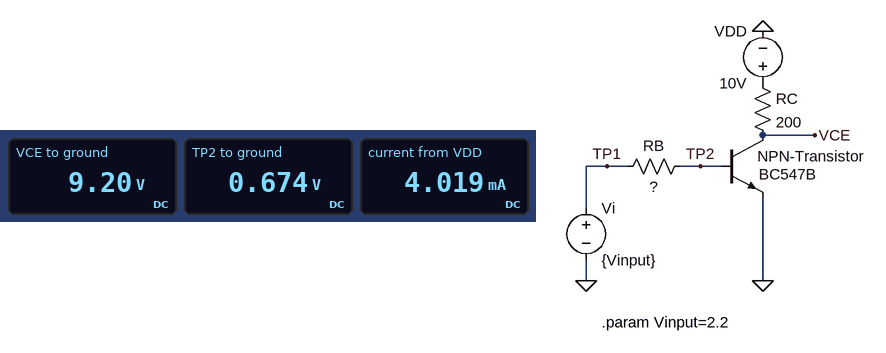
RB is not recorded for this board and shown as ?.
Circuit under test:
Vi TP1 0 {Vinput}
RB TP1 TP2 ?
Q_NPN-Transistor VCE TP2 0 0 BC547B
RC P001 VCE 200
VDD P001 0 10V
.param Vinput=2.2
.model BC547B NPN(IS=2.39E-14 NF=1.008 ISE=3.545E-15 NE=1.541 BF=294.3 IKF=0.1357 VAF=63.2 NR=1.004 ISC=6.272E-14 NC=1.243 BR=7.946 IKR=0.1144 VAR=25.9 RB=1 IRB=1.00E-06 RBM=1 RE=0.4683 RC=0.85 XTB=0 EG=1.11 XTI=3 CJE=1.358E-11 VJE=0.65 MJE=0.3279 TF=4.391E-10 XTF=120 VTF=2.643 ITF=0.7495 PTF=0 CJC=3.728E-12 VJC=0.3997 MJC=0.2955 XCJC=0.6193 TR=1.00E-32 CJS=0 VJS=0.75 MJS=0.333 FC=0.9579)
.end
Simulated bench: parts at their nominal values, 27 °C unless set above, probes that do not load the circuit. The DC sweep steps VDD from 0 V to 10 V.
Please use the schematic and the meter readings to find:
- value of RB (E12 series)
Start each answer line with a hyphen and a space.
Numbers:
- 120 kΩ
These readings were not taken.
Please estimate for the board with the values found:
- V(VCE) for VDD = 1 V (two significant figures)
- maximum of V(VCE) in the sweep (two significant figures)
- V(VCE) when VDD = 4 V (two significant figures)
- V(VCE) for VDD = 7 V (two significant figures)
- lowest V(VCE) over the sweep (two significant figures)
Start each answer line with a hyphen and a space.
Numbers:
- 300 mV
- 9.2 V
- 3.3 V
- 6.2 V
- 2.5 mV
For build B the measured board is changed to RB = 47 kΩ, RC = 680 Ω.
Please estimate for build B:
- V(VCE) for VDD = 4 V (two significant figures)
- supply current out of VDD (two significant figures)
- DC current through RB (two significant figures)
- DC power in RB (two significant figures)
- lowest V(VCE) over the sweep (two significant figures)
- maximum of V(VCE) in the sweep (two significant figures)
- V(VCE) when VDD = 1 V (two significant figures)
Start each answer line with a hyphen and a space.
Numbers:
- 130 mV
- 9.0 mA
- 32 µA
- 48 µW
- 5.4 mV
- 3.9 V
- 63 mV
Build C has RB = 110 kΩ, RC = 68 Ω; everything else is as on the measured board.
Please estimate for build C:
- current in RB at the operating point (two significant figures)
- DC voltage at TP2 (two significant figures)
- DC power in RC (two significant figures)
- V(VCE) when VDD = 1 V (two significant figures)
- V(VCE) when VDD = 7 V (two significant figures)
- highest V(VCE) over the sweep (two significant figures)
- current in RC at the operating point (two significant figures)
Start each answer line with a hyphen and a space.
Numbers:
- 14 µA
- 680 mV
- 1.3 mW
- 740 mV
- 6.7 V
- 9.7 V
- 4.4 mA
